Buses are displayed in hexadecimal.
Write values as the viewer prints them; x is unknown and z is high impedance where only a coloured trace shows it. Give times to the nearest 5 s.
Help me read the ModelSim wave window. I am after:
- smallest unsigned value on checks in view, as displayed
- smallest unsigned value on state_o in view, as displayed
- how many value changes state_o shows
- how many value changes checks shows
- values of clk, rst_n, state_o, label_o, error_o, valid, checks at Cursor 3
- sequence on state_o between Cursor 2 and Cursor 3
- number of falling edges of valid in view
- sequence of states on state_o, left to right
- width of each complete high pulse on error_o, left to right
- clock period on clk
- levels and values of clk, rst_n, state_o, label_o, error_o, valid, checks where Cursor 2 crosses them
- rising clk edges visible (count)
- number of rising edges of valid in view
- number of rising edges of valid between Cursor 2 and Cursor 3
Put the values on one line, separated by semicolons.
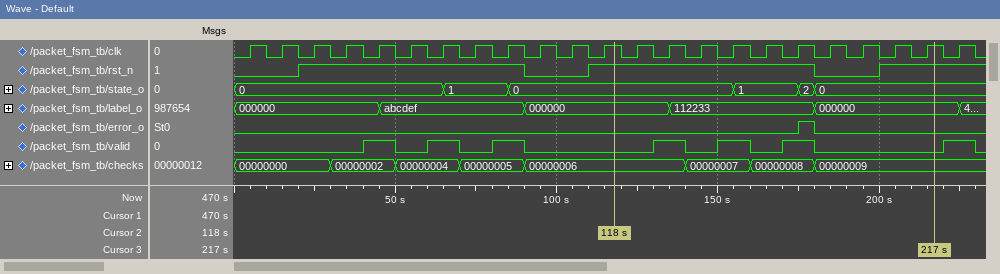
00000000; 0; 5; 7; clk=1, rst_n=1, state_o=0, label_o=000000, error_o=0, valid=0, checks=00000009; 0, 1, 2, 0; 7; 0, 1, 0, 1, 2, 0; 5 s; 10 s; clk=1, rst_n=1, state_o=0, label_o=000000, error_o=0, valid=0, checks=00000006; 23; 7; 3
